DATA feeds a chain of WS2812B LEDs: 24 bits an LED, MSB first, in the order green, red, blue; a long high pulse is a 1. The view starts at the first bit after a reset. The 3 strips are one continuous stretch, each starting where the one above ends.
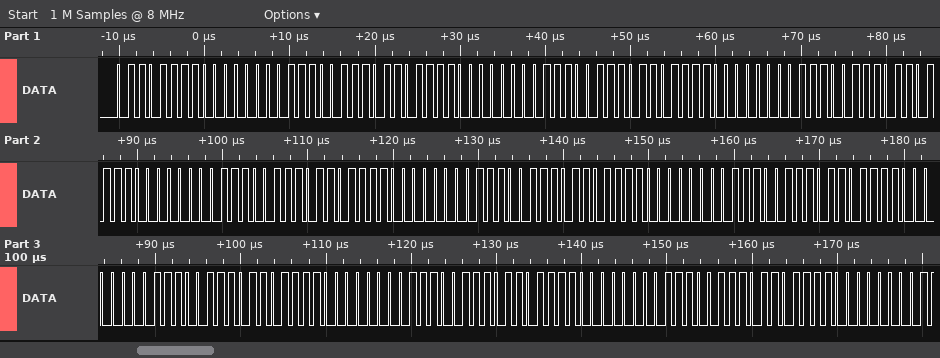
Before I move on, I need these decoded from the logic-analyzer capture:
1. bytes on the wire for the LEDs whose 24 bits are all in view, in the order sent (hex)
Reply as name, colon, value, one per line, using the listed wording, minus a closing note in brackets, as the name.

bytes on the wire for the LEDs whose 24 bits are all in view, in the order sent: 6F 00 E7 6F 00 E7 6F 00 E7 6F 00 E7 6F 00 E7 6F 00 E7 6F 00 E7 6F 00 E7 6F 00 E7
